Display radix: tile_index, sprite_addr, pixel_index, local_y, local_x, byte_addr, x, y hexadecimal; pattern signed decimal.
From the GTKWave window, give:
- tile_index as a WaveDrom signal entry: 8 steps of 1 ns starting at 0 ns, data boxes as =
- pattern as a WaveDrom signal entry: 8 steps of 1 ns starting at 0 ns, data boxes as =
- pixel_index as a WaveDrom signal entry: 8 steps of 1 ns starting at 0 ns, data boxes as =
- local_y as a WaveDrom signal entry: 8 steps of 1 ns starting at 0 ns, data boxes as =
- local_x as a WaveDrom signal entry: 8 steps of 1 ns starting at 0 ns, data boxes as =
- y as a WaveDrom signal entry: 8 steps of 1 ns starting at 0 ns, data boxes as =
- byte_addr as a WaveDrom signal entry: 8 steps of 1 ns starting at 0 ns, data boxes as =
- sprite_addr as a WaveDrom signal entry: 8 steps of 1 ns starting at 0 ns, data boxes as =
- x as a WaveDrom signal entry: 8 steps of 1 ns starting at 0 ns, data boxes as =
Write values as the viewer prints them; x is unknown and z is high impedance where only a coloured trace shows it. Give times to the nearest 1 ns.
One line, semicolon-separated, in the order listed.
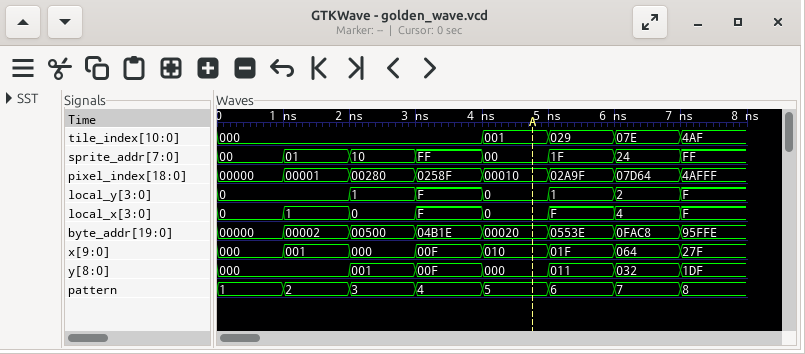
{name: 'tile_index', wave: '=...====', data: '000 001 029 07E 4AF'}; {name: 'pattern', wave: '========', data: '1 2 3 4 5 6 7 8'}; {name: 'pixel_index', wave: '========', data: '00000 00001 00280 0258F 00010 02A9F 07D64 4AFFF'}; {name: 'local_y', wave: '=.======', data: '0 1 F 0 1 2 F'}; {name: 'local_x', wave: '========', data: '0 1 0 F 0 F 4 F'}; {name: 'y', wave: '=.======', data: '000 001 00F 000 011 032 1DF'}; {name: 'byte_addr', wave: '========', data: '00000 00002 00500 04B1E 00020 0553E 0FAC8 95FFE'}; {name: 'sprite_addr', wave: '========', data: '00 01 10 FF 00 1F 24 FF'}; {name: 'x', wave: '========', data: '000 001 000 00F 010 01F 064 27F'}
